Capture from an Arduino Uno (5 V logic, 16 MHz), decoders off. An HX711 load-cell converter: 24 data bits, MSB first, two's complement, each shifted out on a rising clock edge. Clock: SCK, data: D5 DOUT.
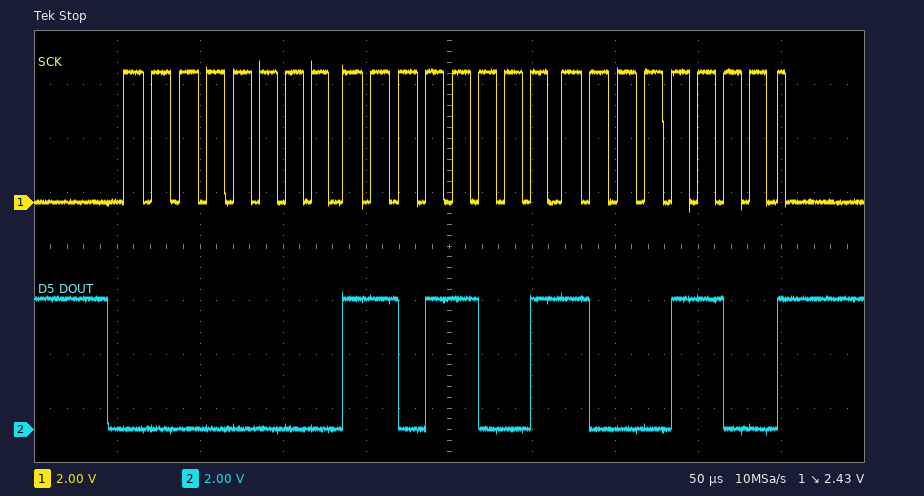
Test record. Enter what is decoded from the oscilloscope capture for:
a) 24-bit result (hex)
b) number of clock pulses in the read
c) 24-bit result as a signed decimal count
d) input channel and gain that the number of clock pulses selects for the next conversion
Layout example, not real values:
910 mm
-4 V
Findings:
0x00D98C
25
55692
channel A, gain 128
